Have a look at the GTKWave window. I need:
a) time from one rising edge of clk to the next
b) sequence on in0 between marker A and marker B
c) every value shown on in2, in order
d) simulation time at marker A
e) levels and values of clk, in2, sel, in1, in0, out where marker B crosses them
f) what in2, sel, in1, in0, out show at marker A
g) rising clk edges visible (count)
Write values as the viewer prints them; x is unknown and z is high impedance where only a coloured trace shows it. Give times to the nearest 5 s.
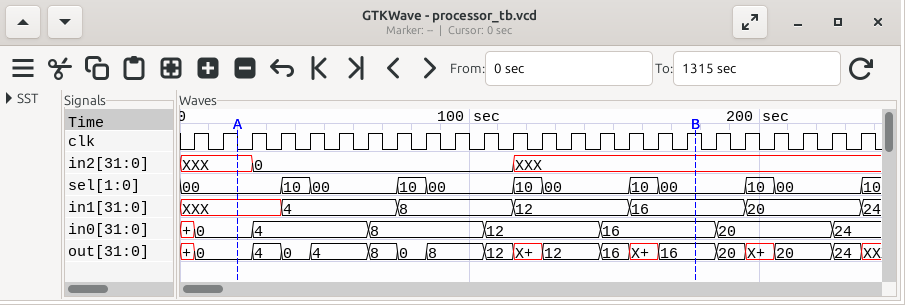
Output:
10 s
0, 4, 8, 12, 16
XXX, 0, XXX
20 s
clk=1, in2=XXX, sel=00, in1=16, in0=16, out=16
in2=XXX, sel=00, in1=XXX, in0=0, out=0
24
